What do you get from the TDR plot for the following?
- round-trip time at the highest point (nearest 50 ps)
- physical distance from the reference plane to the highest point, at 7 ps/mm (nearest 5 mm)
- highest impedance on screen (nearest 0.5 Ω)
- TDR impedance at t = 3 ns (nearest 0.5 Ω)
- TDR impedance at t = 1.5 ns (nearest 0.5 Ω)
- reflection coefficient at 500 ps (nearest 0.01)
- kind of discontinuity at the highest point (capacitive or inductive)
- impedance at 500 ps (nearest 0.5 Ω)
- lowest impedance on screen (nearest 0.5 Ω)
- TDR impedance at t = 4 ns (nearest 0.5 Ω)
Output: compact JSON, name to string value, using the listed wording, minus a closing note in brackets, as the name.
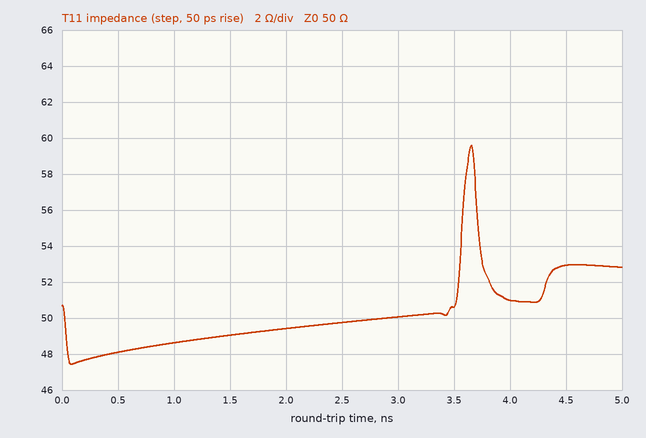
{"round-trip time at the highest point": "3.65 ns", "physical distance from the reference plane to the highest point, at 7 ps/mm": "260 mm", "highest impedance on screen": "59.5 Ω", "TDR impedance at t = 3 ns": "50.0 Ω", "TDR impedance at t = 1.5 ns": "49.0 Ω", "reflection coefficient at 500 ps": "-0.02", "kind of discontinuity at the highest point": "inductive", "impedance at 500 ps": "48.0 Ω", "lowest impedance on screen": "47.5 Ω", "TDR impedance at t = 4 ns": "51.0 Ω"}
